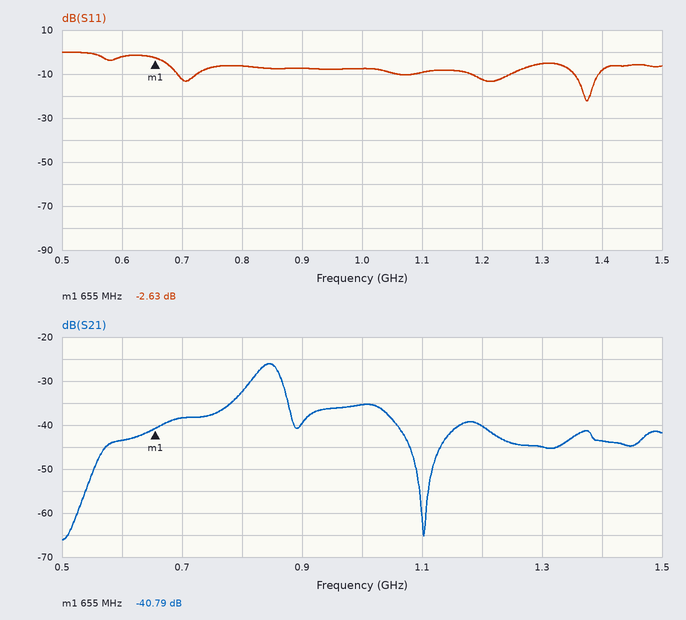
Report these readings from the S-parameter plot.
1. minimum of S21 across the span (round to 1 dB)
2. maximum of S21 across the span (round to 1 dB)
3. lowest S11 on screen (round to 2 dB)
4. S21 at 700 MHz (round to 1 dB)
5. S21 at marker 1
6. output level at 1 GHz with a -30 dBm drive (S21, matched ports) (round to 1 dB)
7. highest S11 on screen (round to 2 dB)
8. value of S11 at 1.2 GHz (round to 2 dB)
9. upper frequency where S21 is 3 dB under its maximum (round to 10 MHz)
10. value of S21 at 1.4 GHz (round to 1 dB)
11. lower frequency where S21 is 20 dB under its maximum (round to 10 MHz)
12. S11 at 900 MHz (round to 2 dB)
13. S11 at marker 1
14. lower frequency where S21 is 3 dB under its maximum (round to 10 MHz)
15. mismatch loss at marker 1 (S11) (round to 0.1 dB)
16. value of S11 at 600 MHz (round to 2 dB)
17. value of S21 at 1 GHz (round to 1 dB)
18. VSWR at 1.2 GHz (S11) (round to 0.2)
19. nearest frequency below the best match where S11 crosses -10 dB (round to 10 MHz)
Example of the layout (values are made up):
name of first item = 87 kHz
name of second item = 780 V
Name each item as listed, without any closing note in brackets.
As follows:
minimum of S21 across the span = -66 dB
maximum of S21 across the span = -26 dB
lowest S11 on screen = -22 dB
S21 at 700 MHz = -38 dB
S21 at marker 1 = -40.79 dB
output level at 1 GHz with a -30 dBm drive (S21, matched ports) = -65 dBm
highest S11 on screen = 0 dB
value of S11 at 1.2 GHz = -12 dB
upper frequency where S21 is 3 dB under its maximum = 860 MHz
value of S21 at 1.4 GHz = -44 dB
lower frequency where S21 is 20 dB under its maximum = 570 MHz
S11 at 900 MHz = -8 dB
S11 at marker 1 = -2.63 dB
lower frequency where S21 is 3 dB under its maximum = 820 MHz
mismatch loss at marker 1 (S11) = 3.4 dB
value of S11 at 600 MHz = -2 dB
value of S21 at 1 GHz = -35 dB
VSWR at 1.2 GHz (S11) = 1.6
nearest frequency below the best match where S11 crosses -10 dB = 1.35 GHz
